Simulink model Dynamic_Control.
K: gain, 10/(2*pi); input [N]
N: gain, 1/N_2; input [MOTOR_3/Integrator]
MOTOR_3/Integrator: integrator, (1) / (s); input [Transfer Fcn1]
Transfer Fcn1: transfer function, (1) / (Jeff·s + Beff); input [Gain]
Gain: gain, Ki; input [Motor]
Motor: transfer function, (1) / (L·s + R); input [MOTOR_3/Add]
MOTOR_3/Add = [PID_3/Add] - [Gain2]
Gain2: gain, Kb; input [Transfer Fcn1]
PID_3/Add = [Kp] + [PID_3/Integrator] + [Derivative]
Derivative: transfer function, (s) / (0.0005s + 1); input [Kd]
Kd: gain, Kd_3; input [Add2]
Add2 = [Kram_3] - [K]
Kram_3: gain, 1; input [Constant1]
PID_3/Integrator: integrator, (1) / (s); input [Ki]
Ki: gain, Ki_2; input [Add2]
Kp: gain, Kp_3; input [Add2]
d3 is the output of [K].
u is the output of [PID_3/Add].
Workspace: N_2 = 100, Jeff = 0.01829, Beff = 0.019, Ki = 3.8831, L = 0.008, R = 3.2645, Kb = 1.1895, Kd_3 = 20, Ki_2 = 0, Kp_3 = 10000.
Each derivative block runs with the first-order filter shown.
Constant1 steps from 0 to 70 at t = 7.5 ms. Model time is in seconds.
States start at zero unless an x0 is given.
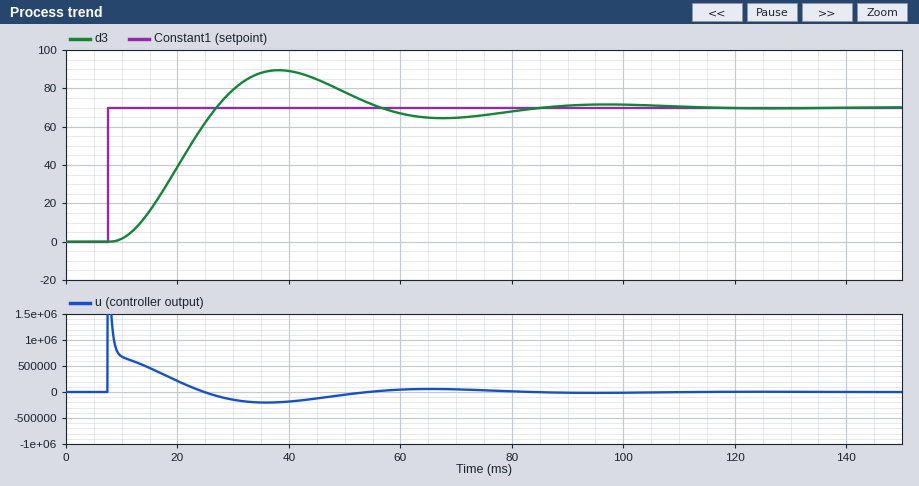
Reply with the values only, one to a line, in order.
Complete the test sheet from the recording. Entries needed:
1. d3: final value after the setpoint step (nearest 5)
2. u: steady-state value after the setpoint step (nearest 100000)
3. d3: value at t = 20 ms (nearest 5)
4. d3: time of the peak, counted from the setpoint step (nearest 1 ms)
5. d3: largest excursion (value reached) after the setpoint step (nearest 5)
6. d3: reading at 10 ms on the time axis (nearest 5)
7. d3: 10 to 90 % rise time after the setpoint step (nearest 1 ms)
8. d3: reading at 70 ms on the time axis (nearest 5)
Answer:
70
0
40
31 ms
90
0
13 ms
65
